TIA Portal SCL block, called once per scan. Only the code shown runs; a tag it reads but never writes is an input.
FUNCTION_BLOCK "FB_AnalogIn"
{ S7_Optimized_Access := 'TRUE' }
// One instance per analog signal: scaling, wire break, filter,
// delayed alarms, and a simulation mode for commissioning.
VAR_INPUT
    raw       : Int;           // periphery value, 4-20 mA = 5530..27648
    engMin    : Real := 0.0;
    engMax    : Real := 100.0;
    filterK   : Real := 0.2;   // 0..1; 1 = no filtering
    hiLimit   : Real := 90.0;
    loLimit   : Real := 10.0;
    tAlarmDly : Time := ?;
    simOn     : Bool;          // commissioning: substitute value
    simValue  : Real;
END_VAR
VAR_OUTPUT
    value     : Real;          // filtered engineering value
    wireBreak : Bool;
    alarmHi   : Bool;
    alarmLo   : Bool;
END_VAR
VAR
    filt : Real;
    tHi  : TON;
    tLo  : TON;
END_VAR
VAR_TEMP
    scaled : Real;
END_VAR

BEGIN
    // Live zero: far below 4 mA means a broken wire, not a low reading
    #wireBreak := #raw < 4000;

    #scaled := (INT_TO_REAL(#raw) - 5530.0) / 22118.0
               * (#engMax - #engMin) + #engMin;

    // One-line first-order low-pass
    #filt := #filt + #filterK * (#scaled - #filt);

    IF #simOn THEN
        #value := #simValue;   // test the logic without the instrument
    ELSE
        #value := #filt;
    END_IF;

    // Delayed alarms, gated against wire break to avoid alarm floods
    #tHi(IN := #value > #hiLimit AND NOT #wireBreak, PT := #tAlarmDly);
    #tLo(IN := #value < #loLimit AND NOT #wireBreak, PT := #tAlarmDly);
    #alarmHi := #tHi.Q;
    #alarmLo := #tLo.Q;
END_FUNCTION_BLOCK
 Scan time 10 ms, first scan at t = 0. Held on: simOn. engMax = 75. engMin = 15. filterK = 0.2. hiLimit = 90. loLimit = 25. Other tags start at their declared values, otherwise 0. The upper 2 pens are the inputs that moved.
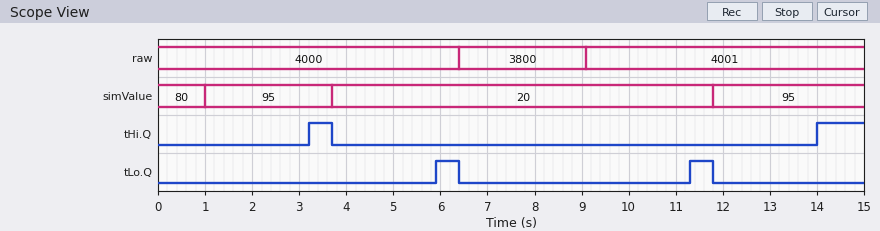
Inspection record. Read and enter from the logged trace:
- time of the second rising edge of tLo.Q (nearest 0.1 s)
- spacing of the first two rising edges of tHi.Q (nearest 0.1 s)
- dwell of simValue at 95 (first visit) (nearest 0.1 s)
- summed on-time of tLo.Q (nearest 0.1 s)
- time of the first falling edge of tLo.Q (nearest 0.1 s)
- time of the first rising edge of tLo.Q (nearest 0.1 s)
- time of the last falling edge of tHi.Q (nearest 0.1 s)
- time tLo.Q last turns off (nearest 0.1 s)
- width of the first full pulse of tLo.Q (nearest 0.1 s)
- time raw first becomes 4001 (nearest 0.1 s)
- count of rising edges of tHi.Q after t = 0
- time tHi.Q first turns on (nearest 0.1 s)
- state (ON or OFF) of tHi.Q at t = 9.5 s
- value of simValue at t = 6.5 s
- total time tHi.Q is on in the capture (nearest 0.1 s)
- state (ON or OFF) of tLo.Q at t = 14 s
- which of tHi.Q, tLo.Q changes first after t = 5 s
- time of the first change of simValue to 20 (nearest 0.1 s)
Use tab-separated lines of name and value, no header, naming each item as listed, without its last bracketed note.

time of the second rising edge of tLo.Q	11.3 s
spacing of the first two rising edges of tHi.Q	10.8 s
dwell of simValue at 95 (first visit)	2.7 s
summed on-time of tLo.Q	1.0 s
time of the first falling edge of tLo.Q	6.4 s
time of the first rising edge of tLo.Q	5.9 s
time of the last falling edge of tHi.Q	3.7 s
time tLo.Q last turns off	11.8 s
width of the first full pulse of tLo.Q	0.5 s
time raw first becomes 4001	9.1 s
count of rising edges of tHi.Q after t = 0	2
time tHi.Q first turns on	3.2 s
state (ON or OFF) of tHi.Q at t = 9.5 s	OFF
value of simValue at t = 6.5 s	20
total time tHi.Q is on in the capture	1.5 s
state (ON or OFF) of tLo.Q at t = 14 s	OFF
which of tHi.Q, tLo.Q changes first after t = 5 s	tLo.Q
time of the first change of simValue to 20	3.7 s
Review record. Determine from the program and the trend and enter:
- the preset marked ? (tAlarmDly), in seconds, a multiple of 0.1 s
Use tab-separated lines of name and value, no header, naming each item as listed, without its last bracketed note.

the preset marked ? (tAlarmDly), in seconds, a multiple of 0.1 s	2.2 s
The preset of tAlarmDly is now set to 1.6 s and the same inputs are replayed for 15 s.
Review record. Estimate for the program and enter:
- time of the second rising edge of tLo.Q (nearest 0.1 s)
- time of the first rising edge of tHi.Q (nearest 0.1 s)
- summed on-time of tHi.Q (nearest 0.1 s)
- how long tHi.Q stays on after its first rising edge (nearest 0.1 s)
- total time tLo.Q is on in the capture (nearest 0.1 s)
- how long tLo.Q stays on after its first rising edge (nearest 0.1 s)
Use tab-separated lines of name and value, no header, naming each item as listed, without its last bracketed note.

time of the second rising edge of tLo.Q	10.7 s
time of the first rising edge of tHi.Q	2.6 s
summed on-time of tHi.Q	2.7 s
how long tHi.Q stays on after its first rising edge	1.1 s
total time tLo.Q is on in the capture	2.2 s
how long tLo.Q stays on after its first rising edge	1.1 s
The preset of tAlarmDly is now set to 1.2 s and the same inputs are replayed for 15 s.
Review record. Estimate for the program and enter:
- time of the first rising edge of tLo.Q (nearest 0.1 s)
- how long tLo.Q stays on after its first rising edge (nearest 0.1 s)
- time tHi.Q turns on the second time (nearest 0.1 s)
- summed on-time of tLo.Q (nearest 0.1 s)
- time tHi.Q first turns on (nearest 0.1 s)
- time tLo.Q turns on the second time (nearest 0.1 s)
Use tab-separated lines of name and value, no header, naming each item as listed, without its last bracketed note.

time of the first rising edge of tLo.Q	4.9 s
how long tLo.Q stays on after its first rising edge	1.5 s
time tHi.Q turns on the second time	13.0 s
summed on-time of tLo.Q	3.0 s
time tHi.Q first turns on	2.2 s
time tLo.Q turns on the second time	10.3 s
